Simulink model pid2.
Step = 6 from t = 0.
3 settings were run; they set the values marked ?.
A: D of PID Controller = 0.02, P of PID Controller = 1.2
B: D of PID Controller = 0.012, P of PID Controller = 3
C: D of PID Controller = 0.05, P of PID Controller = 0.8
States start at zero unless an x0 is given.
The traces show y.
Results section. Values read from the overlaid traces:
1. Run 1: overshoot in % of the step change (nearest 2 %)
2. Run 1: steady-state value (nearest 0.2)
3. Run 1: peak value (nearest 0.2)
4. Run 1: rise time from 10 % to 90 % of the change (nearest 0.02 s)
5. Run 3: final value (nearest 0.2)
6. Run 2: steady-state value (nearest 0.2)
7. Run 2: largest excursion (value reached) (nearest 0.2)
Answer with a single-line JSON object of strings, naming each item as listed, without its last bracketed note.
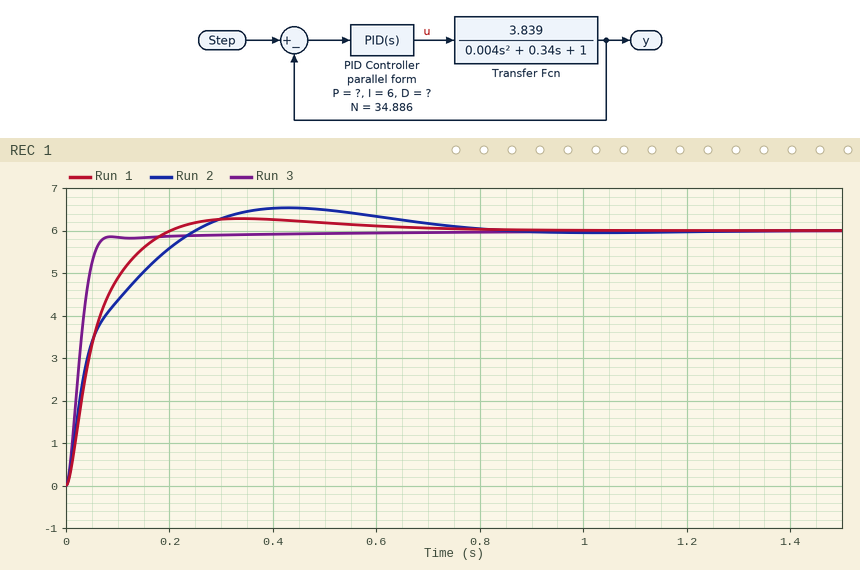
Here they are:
{"Run 1: overshoot in % of the step change": "4 %", "Run 1: steady-state value": "6.0", "Run 1: peak value": "6.2", "Run 1: rise time from 10 % to 90 % of the change": "0.12 s", "Run 3: final value": "6.0", "Run 2: steady-state value": "6.0", "Run 2: largest excursion (value reached)": "6.6"}
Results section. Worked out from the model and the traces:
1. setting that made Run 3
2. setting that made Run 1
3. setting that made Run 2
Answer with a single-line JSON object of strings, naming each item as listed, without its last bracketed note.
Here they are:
{"setting that made Run 3": "B", "setting that made Run 1": "A", "setting that made Run 2": "C"}
